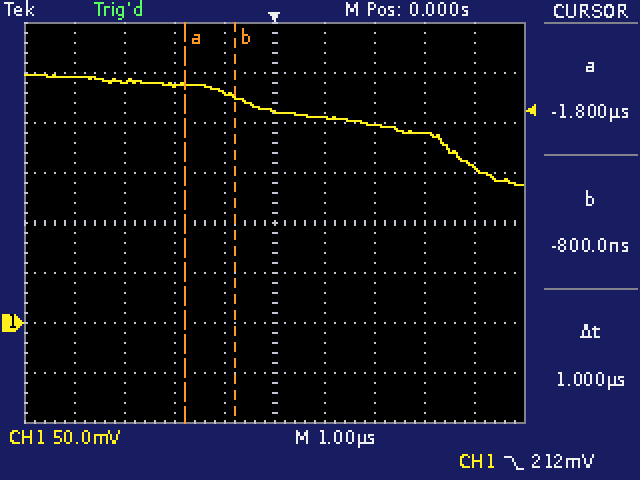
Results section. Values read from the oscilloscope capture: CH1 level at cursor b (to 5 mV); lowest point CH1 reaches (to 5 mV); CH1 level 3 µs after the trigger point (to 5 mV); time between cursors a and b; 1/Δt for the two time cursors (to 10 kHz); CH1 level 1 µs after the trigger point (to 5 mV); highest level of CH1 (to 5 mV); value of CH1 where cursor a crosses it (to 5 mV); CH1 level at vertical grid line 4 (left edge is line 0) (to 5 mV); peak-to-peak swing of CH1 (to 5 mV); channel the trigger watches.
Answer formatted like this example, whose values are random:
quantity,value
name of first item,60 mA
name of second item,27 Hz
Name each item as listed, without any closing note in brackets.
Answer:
quantity,value
CH1 level at cursor b,225 mV
lowest point CH1 reaches,140 mV
CH1 level 3 µs after the trigger point,190 mV
time between cursors a and b,1 µs
1/Δt for the two time cursors,1.00 MHz
CH1 level 1 µs after the trigger point,205 mV
highest level of CH1,250 mV
value of CH1 where cursor a crosses it,240 mV
CH1 level at vertical grid line 4 (left edge is line 0),230 mV
peak-to-peak swing of CH1,110 mV
channel the trigger watches,CH1
